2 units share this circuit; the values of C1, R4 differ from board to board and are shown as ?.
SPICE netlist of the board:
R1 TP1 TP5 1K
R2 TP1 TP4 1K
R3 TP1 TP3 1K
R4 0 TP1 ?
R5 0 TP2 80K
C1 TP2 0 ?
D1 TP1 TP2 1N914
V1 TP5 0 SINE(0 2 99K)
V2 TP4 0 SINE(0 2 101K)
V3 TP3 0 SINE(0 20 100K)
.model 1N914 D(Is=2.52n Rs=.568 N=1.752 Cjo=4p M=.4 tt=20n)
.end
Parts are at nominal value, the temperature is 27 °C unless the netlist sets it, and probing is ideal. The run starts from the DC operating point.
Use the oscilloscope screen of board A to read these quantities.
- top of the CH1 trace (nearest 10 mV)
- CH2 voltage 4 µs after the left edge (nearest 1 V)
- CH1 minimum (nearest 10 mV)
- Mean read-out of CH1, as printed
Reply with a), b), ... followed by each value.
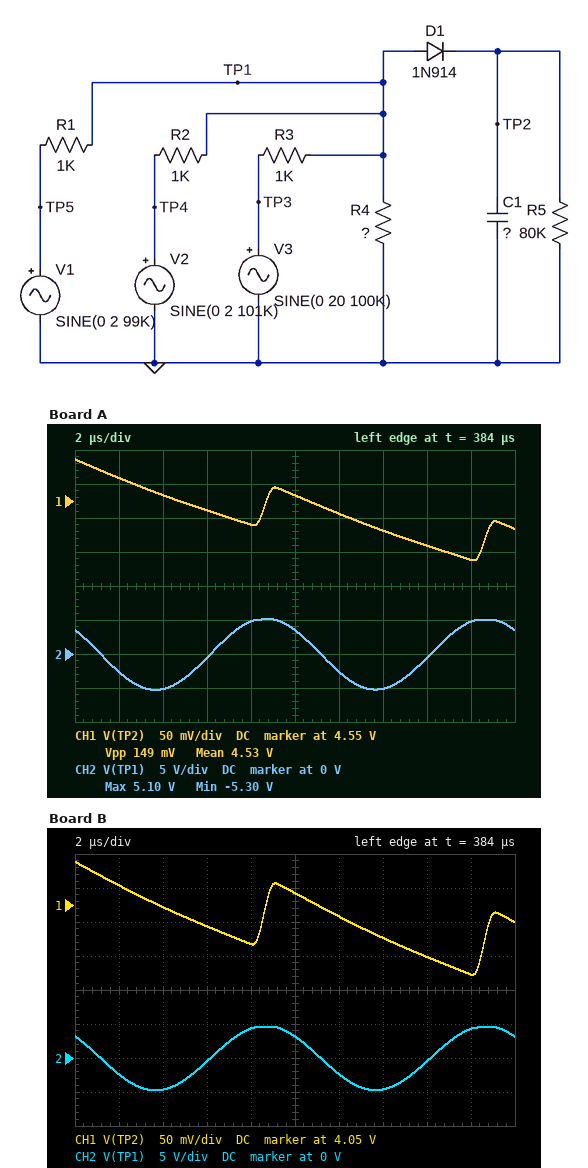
a) 4.61 V
b) -5 V
c) 4.46 V
d) 4.53 V
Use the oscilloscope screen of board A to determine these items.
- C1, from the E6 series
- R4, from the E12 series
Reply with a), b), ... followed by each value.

a) 4.7 nF
b) 4.7 kΩ
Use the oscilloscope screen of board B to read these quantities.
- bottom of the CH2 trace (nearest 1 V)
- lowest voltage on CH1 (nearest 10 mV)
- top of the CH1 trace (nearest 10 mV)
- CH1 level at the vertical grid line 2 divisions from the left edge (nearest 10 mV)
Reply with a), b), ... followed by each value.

a) -5 V
b) 3.95 V
c) 4.11 V
d) 4.05 V
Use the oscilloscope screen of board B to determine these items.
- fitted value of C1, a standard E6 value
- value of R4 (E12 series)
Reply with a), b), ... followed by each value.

a) 3.3 nF
b) 1.8 kΩ
